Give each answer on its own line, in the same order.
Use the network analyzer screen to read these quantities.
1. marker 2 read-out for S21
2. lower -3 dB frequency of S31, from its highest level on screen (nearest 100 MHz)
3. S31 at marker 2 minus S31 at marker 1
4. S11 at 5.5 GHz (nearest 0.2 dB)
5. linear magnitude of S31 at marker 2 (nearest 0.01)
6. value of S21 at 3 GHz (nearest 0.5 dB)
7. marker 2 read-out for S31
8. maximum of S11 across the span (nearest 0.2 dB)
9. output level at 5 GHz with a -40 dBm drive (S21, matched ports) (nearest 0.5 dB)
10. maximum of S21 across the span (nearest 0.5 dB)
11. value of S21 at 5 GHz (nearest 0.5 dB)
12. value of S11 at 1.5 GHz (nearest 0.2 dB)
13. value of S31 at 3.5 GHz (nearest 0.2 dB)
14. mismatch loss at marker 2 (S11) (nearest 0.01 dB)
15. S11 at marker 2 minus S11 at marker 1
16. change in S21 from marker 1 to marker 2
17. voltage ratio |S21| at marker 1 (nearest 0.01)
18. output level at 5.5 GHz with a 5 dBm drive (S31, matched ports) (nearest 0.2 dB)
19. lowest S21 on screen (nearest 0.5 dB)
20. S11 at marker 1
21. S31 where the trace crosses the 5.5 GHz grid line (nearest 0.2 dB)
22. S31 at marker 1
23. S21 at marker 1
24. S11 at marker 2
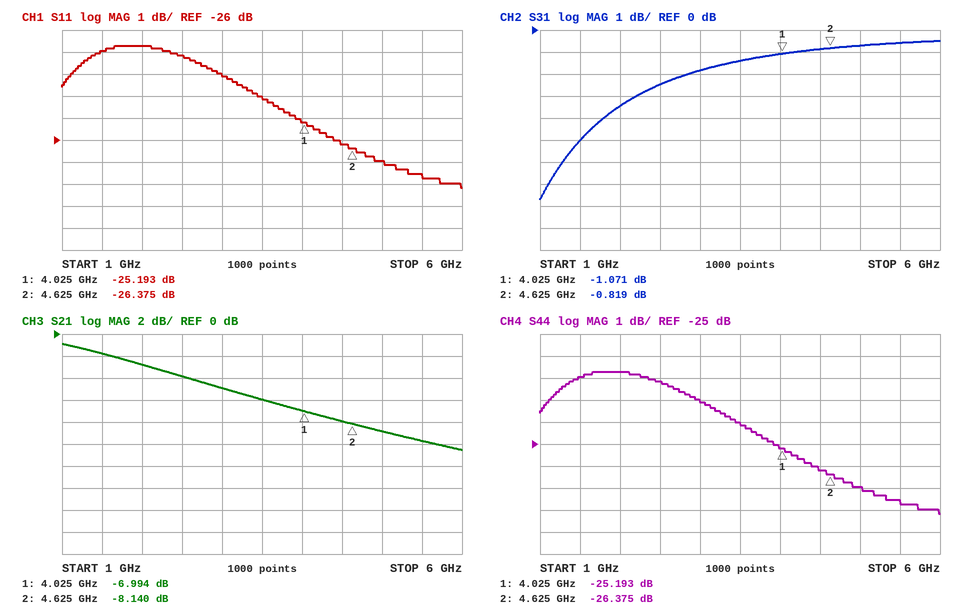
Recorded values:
-8.140 dB
2.0 GHz
0.252 dB
-27.6 dB
0.91
-5.0 dB
-0.819 dB
-21.8 dB
-49.0 dBm
-1.0 dB
-9.0 dB
-22.0 dB
-1.4 dB
0.01 dB
-1.182 dB
-1.146 dB
0.45
4.4 dBm
-10.5 dB
-25.193 dB
-0.6 dB
-1.071 dB
-6.994 dB
-26.375 dB
